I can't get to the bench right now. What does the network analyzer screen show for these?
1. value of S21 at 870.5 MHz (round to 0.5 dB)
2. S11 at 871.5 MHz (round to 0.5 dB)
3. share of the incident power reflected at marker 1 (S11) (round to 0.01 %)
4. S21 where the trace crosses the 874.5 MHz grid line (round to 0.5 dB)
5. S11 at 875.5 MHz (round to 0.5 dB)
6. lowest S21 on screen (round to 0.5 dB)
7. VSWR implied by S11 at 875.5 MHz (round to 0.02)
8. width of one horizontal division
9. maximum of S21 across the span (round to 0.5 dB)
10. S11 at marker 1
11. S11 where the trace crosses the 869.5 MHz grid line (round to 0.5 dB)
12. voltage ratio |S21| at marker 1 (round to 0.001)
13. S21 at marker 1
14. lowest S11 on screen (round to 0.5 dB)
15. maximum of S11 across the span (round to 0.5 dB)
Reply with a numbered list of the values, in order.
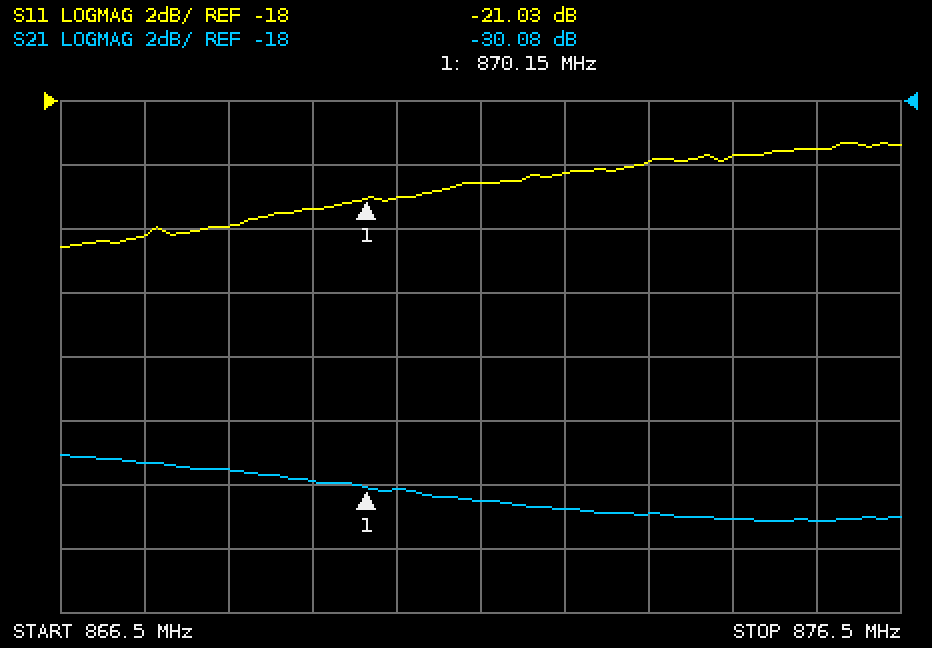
1. -30.0 dB
2. -20.5 dB
3. 0.79 %
4. -31.0 dB
5. -19.5 dB
6. -31.0 dB
7. 1.24
8. 1 MHz
9. -29.0 dB
10. -21.03 dB
11. -21.5 dB
12. 0.031
13. -30.08 dB
14. -22.5 dB
15. -19.5 dB
